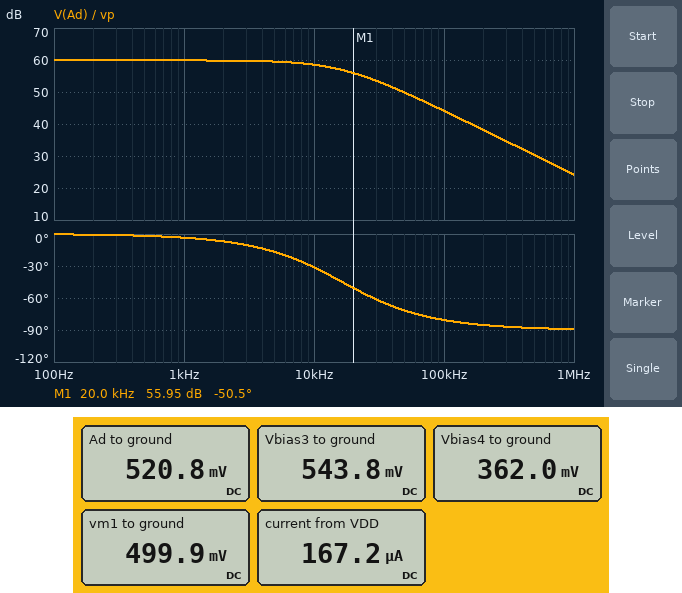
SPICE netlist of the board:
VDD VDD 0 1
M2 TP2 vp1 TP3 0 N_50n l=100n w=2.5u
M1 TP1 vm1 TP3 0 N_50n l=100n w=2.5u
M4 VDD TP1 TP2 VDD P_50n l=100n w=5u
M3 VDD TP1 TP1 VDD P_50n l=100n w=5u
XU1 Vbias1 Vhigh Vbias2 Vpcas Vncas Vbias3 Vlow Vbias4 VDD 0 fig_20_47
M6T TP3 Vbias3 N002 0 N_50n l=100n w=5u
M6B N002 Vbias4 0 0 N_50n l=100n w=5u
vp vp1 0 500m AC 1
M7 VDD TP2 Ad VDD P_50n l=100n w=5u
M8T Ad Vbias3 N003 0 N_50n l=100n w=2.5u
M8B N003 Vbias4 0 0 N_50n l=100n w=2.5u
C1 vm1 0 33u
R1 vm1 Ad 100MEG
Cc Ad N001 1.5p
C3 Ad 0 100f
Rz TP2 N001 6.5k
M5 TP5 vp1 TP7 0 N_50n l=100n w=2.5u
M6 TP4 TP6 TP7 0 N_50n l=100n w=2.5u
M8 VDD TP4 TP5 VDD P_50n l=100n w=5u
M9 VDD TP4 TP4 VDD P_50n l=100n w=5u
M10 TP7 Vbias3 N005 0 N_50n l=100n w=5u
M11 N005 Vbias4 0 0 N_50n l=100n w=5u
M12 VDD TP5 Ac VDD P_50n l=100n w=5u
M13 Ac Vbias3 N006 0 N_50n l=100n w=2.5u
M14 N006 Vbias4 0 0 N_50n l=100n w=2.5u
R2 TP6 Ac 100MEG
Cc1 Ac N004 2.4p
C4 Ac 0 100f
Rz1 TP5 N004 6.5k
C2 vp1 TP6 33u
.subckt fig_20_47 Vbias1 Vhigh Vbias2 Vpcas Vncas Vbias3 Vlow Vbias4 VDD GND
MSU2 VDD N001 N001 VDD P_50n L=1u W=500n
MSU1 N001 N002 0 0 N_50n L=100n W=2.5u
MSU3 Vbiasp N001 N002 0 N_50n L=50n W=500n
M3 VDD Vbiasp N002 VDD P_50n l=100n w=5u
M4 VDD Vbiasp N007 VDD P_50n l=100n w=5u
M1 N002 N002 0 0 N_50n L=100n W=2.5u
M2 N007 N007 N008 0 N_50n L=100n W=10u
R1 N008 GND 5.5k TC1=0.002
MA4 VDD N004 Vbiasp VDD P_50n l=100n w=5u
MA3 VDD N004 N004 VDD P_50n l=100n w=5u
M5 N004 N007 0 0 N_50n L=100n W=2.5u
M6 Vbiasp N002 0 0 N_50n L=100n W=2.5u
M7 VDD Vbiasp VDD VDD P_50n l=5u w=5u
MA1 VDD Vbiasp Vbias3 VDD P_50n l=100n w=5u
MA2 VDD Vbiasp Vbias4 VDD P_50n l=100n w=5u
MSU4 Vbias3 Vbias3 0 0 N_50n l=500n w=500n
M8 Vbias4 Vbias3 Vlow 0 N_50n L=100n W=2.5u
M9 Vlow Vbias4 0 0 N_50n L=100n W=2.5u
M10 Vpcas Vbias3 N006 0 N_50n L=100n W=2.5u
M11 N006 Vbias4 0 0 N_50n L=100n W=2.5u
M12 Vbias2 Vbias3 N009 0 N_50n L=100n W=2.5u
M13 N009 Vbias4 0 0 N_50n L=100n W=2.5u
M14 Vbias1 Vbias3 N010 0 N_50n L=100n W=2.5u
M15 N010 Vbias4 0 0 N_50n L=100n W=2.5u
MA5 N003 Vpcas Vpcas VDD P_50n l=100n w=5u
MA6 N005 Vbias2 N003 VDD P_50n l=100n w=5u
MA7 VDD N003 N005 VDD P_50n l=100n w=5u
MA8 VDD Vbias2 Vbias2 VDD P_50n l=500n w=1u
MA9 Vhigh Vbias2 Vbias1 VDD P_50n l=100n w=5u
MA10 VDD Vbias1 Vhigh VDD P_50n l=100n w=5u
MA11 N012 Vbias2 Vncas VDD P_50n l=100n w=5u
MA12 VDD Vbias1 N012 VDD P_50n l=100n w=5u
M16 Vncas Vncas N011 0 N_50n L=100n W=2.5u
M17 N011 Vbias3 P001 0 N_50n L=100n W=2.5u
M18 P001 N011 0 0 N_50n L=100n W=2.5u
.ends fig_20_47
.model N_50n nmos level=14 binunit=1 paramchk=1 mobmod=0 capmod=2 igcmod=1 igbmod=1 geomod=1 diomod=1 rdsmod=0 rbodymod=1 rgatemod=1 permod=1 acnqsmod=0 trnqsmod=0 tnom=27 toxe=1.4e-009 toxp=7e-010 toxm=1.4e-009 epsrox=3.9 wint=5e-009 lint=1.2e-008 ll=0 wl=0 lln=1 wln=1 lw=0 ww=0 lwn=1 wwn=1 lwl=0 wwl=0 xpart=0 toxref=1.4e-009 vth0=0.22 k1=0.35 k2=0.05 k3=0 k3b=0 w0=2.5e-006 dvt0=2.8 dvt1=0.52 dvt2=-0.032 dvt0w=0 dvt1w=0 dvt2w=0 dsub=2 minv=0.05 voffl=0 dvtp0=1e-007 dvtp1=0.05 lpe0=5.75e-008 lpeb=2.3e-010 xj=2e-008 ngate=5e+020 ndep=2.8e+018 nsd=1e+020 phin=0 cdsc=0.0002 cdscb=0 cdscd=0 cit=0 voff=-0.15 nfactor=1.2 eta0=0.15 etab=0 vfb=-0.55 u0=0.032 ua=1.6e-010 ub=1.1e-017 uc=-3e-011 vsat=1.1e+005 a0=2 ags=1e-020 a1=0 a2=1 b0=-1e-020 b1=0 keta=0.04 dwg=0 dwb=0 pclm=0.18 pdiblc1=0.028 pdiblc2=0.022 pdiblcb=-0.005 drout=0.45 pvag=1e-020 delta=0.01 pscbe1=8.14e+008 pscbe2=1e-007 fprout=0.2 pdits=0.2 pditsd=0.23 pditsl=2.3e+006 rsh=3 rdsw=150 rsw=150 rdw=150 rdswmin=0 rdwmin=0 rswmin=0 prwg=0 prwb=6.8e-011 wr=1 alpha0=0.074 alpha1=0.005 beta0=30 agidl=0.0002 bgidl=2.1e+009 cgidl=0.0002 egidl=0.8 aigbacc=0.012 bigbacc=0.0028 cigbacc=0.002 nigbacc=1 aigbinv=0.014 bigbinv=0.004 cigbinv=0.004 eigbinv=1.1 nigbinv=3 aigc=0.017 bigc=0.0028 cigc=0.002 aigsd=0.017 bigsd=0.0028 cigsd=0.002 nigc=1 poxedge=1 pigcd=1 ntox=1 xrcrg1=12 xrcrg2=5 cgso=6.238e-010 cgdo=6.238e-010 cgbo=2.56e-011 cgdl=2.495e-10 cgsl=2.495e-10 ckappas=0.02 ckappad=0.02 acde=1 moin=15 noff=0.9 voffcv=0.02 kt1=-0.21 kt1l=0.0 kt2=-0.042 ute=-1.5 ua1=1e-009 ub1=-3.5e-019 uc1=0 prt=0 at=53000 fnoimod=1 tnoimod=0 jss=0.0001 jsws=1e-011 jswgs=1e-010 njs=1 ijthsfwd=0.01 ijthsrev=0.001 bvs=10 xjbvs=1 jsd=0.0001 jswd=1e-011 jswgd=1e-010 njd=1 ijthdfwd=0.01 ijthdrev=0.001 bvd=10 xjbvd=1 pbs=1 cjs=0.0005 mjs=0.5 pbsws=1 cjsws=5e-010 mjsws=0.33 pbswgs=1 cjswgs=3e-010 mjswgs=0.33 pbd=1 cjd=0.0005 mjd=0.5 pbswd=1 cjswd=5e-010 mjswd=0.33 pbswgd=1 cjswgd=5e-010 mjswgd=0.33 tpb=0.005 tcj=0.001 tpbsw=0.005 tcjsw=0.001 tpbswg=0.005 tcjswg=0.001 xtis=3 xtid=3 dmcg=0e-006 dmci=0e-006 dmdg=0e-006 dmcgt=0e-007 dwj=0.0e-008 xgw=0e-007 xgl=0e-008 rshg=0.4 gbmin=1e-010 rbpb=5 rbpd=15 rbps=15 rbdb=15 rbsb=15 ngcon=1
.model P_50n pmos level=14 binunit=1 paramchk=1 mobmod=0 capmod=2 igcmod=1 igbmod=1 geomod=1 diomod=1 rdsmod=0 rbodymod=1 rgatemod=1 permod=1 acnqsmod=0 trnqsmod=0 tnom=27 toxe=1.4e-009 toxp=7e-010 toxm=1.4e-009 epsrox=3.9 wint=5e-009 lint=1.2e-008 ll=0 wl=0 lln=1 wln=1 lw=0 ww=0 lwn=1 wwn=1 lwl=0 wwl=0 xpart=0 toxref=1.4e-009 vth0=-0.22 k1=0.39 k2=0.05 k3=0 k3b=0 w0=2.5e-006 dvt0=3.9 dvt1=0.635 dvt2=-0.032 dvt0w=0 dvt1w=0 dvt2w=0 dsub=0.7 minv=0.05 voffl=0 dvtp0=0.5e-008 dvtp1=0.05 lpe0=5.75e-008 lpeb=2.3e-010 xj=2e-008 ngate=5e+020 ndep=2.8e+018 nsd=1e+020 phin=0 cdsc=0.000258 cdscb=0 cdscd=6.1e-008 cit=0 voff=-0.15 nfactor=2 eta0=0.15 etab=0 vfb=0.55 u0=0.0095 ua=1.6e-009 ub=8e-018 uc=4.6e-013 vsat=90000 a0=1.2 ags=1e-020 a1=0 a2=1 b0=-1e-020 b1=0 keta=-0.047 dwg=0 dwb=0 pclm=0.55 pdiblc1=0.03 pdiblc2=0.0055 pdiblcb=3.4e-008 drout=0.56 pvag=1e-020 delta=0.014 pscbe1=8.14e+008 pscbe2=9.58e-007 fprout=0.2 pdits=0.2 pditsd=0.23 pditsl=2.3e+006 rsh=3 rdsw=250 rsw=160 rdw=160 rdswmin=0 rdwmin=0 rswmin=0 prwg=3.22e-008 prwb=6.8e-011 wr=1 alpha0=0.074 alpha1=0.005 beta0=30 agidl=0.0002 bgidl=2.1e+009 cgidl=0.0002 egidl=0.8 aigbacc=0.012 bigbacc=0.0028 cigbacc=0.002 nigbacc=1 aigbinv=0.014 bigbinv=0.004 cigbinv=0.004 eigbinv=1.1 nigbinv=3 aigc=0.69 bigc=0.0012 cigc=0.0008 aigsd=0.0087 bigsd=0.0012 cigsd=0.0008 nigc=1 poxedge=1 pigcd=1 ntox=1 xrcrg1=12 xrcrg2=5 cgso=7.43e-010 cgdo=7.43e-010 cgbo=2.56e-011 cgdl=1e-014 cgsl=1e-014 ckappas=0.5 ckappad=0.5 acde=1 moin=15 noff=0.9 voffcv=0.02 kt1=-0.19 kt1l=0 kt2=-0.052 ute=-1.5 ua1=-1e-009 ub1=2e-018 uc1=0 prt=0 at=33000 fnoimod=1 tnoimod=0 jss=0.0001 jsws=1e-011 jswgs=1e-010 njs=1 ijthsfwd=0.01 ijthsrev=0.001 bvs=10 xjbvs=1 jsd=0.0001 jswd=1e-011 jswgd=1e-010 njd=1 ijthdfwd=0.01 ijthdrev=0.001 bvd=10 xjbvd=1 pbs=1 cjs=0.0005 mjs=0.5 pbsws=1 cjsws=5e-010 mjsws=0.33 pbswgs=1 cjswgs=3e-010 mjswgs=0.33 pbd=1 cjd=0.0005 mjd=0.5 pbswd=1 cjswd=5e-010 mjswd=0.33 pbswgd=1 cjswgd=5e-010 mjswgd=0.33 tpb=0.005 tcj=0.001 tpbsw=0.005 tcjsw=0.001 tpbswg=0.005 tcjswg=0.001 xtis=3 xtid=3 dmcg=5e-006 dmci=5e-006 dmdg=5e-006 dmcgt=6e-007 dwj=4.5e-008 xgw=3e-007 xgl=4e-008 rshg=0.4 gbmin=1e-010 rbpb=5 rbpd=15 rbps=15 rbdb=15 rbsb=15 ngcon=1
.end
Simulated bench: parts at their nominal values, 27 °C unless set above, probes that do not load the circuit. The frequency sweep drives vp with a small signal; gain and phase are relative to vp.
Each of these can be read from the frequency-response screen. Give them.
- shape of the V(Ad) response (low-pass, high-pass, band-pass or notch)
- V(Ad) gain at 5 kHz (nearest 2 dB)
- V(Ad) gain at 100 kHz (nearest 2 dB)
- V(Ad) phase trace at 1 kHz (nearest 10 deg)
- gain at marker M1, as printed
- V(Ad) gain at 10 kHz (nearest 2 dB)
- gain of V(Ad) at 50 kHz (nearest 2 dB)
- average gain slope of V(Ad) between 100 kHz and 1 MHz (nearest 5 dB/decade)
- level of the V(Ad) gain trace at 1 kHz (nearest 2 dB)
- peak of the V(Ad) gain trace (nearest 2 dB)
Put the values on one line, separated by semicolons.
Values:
low-pass; 60 dB; 44 dB; 0 deg; 55.95 dB; 58 dB; 50 dB; -20 dB/decade; 60 dB; 60 dB
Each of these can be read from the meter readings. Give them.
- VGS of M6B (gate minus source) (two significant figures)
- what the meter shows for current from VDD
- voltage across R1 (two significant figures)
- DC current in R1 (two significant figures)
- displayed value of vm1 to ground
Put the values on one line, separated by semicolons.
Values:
360 mV; 167.2 µA; 21 mV; 210 pA; 499.9 mV
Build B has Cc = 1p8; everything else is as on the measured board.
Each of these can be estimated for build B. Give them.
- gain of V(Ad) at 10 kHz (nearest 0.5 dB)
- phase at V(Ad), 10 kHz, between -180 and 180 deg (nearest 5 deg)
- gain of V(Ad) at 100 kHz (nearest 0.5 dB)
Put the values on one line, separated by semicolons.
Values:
58.0 dB; -35 deg; 42.5 dB
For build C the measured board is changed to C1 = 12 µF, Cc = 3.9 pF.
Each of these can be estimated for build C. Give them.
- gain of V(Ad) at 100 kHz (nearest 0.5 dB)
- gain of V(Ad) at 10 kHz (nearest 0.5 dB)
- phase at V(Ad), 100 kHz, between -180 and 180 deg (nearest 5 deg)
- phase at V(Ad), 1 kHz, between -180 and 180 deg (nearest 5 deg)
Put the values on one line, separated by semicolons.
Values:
36.0 dB; 54.5 dB; -85 deg; -10 deg
